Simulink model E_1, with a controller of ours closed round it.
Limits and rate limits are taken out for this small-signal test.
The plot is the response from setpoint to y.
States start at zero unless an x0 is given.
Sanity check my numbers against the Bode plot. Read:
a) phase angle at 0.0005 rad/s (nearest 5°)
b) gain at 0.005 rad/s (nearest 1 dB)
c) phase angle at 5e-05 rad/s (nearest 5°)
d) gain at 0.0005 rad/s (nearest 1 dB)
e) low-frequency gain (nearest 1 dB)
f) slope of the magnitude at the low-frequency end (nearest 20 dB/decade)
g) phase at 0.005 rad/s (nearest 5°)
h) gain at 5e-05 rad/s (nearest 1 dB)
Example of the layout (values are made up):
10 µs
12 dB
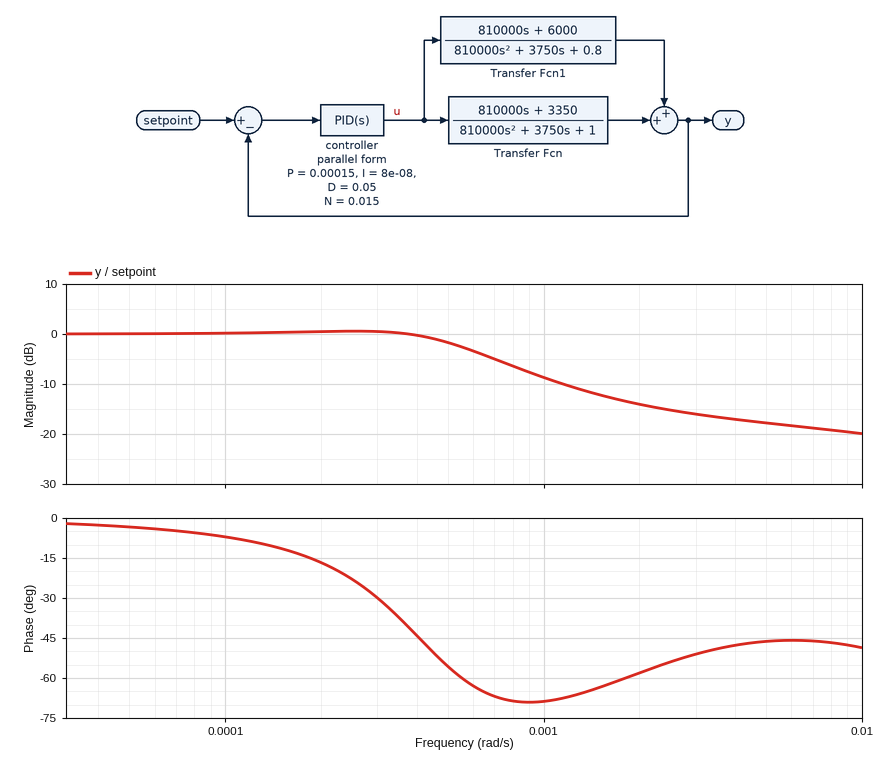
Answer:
-55°
-18 dB
-5°
-2 dB
0 dB
0 dB/decade
-45°
0 dB
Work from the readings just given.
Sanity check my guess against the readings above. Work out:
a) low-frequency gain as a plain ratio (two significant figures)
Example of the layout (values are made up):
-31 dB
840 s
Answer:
1.0
